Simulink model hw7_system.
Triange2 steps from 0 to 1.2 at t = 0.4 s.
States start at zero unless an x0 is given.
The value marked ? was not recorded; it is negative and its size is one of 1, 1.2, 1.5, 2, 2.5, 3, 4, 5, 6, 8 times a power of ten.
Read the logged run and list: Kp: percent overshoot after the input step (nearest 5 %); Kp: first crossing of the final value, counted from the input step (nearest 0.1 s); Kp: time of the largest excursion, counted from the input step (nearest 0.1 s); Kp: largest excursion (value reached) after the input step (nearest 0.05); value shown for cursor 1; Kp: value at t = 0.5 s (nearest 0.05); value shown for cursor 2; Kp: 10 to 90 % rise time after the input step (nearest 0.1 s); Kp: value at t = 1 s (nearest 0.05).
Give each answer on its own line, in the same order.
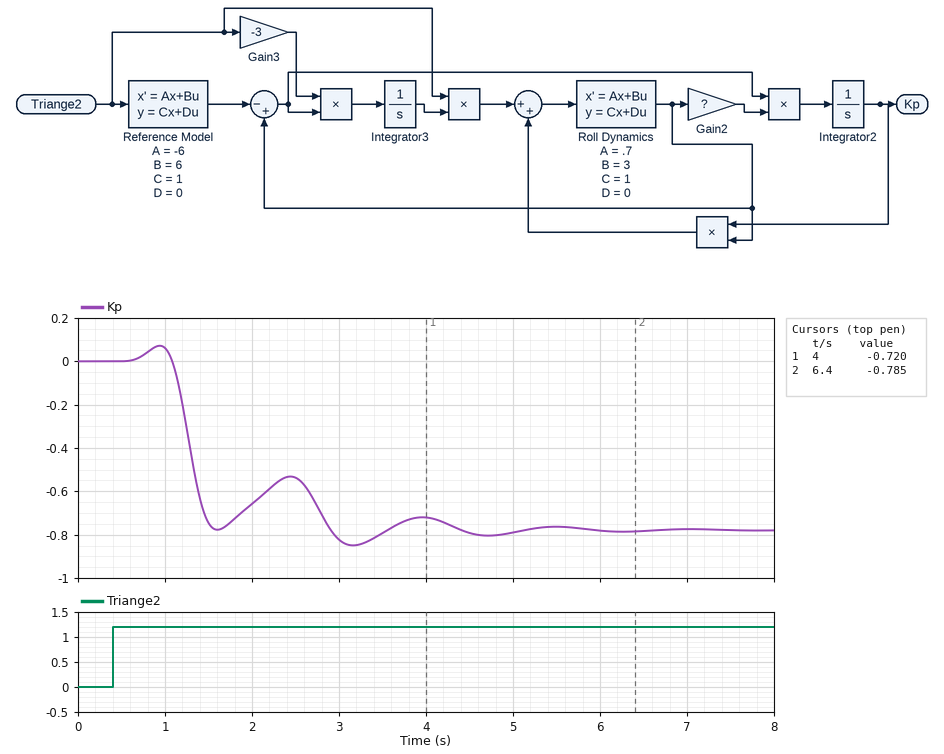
10 %
2.5 s
2.8 s
-0.85
-0.720
0.00
-0.785
0.3 s
0.05
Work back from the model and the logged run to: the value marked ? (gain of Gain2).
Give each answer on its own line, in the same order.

-1
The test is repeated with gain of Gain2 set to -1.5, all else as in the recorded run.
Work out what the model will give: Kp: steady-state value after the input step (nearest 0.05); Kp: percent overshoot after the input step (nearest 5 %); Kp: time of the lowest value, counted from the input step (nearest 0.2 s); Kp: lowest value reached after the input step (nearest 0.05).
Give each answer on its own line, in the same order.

-0.85
10 %
1.2 s
-0.95
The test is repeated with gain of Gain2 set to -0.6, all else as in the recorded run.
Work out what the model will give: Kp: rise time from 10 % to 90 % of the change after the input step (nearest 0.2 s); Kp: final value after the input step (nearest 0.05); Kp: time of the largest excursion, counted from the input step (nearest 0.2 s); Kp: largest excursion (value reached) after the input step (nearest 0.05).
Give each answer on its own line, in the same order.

1.8 s
-0.70
2.8 s
-0.75
